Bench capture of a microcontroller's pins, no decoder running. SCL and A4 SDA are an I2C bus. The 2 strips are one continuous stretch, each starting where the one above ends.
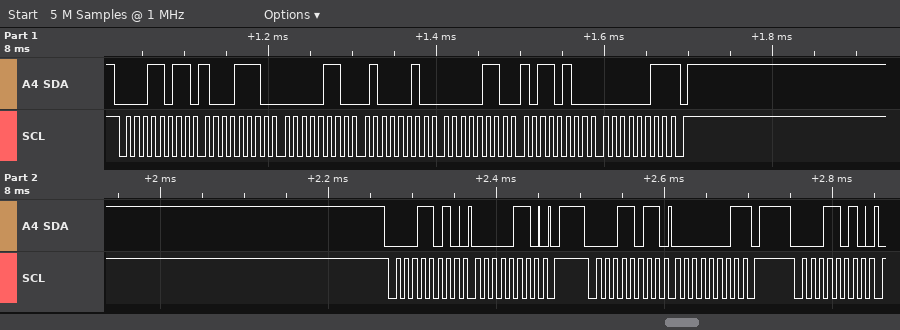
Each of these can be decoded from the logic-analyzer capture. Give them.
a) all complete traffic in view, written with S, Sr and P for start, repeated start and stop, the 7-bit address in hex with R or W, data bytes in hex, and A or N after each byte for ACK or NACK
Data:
S 0DR A 8E A 06 A 42 A 06 A B4 A 03 N P S 0DW A 06 A P S 0DR A 01 N P S 0DW A
